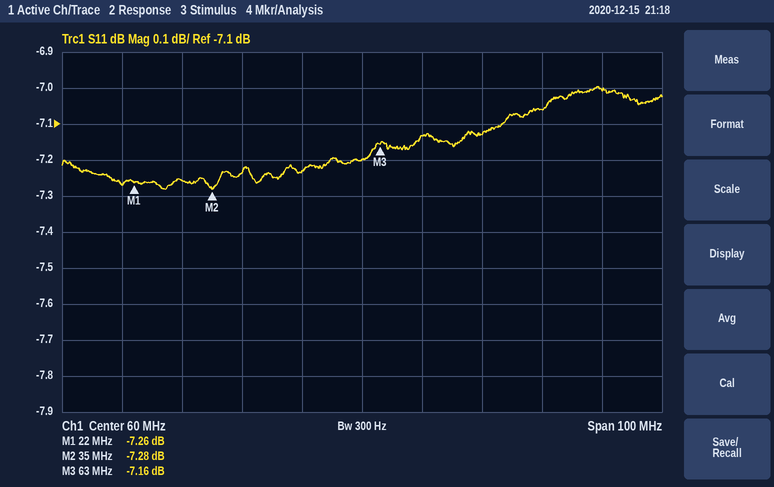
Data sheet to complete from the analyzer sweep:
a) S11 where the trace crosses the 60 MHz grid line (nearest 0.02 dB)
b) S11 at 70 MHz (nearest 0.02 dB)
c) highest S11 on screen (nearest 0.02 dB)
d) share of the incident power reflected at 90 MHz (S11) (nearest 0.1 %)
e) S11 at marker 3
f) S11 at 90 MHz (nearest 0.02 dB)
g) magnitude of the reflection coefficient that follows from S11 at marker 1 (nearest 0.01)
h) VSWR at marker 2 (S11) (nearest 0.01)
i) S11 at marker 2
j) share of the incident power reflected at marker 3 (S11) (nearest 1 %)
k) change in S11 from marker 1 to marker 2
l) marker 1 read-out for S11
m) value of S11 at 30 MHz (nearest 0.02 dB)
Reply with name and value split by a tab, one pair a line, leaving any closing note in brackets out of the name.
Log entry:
S11 where the trace crosses the 60 MHz grid line	-7.20 dB
S11 at 70 MHz	-7.14 dB
highest S11 on screen	-7.00 dB
share of the incident power reflected at 90 MHz (S11)	19.7 %
S11 at marker 3	-7.16 dB
S11 at 90 MHz	-7.06 dB
magnitude of the reflection coefficient that follows from S11 at marker 1	0.43
VSWR at marker 2 (S11)	2.52
S11 at marker 2	-7.28 dB
share of the incident power reflected at marker 3 (S11)	19 %
change in S11 from marker 1 to marker 2	-0.02 dB
marker 1 read-out for S11	-7.26 dB
value of S11 at 30 MHz	-7.26 dB
